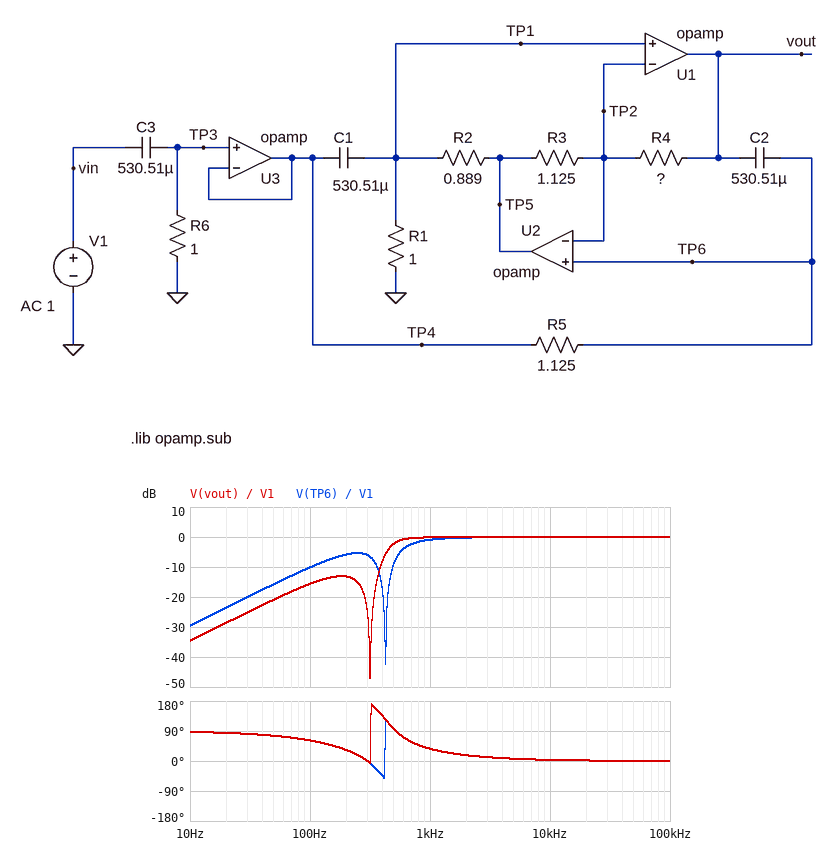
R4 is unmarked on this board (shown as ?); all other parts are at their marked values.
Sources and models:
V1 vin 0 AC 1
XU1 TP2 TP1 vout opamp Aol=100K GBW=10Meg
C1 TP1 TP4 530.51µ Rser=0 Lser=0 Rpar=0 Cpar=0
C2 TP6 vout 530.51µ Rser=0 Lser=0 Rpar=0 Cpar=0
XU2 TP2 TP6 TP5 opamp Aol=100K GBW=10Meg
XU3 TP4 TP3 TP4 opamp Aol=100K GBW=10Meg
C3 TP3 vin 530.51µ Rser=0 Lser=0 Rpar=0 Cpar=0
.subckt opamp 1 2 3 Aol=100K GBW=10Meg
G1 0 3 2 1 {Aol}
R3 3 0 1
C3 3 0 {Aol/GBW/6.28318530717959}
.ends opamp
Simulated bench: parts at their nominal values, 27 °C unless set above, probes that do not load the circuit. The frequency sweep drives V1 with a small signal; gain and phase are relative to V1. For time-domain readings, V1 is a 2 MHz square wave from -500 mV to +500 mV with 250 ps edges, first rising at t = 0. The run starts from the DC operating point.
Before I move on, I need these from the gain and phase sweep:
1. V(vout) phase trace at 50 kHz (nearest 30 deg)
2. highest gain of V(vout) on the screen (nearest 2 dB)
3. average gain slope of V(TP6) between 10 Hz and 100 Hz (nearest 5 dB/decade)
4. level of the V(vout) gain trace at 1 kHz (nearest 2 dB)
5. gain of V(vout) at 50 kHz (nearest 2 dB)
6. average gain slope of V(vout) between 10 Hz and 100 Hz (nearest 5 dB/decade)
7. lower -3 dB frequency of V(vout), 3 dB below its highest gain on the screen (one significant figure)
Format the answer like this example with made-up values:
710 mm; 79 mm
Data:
0 deg; 0 dB; 20 dB/decade; 0 dB; 0 dB; 20 dB/decade; 500 Hz
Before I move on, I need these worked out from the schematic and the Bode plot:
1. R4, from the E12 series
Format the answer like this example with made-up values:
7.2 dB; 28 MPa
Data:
0.56 Ω
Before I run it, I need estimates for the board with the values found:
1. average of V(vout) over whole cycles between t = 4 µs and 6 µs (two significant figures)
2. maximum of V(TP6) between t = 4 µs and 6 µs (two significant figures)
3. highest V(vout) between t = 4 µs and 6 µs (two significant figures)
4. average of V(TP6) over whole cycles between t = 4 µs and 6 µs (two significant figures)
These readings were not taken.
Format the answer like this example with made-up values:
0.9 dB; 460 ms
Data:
490 mV; 1.1 V; 1.1 V; 490 mV
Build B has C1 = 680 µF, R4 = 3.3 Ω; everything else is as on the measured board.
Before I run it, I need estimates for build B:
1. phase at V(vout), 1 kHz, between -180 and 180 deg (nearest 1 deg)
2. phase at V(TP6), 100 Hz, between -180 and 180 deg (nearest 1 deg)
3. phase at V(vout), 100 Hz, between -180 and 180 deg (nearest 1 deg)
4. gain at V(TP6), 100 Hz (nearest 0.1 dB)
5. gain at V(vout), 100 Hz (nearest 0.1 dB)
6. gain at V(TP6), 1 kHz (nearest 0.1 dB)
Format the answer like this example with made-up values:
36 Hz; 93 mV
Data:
30 deg; 12 deg; -168 deg; -15.8 dB; -5.0 dB; -0.6 dB
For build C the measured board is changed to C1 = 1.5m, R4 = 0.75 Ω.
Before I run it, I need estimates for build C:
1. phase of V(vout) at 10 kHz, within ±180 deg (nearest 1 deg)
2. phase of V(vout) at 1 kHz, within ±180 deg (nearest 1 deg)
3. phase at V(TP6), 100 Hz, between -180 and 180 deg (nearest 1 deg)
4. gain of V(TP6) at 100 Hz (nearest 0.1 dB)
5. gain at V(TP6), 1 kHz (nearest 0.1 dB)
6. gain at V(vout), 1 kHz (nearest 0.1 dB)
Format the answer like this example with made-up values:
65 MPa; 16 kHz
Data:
2 deg; 23 deg; 56 deg; -10.3 dB; -0.4 dB; -0.2 dB
